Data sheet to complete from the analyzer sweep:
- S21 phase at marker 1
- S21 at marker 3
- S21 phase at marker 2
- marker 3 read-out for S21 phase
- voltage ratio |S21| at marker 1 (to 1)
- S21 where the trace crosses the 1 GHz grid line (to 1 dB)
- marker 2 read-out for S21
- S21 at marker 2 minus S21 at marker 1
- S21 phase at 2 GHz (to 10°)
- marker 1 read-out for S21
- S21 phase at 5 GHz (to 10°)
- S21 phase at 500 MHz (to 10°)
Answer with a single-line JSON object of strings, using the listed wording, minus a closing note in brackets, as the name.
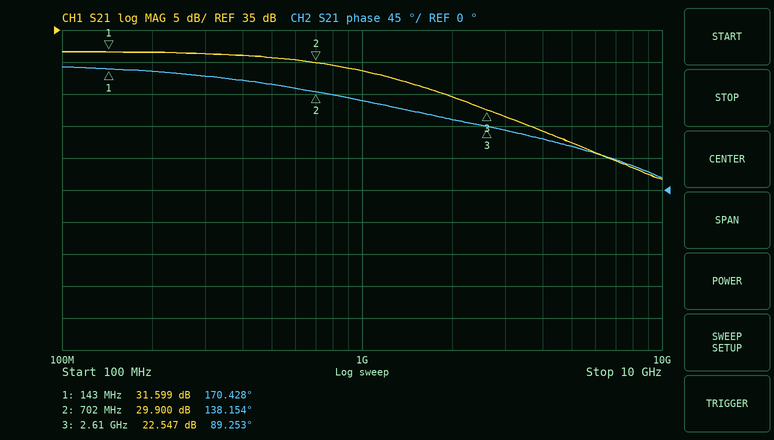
{"S21 phase at marker 1": "170.428°", "S21 at marker 3": "22.547 dB", "S21 phase at marker 2": "138.154°", "marker 3 read-out for S21 phase": "89.253°", "voltage ratio |S21| at marker 1": "38", "S21 where the trace crosses the 1 GHz grid line": "29 dB", "marker 2 read-out for S21": "29.900 dB", "S21 at marker 2 minus S21 at marker 1": "-1.699 dB", "S21 phase at 2 GHz": "100°", "marker 1 read-out for S21": "31.599 dB", "S21 phase at 5 GHz": "60°", "S21 phase at 500 MHz": "150°"}
